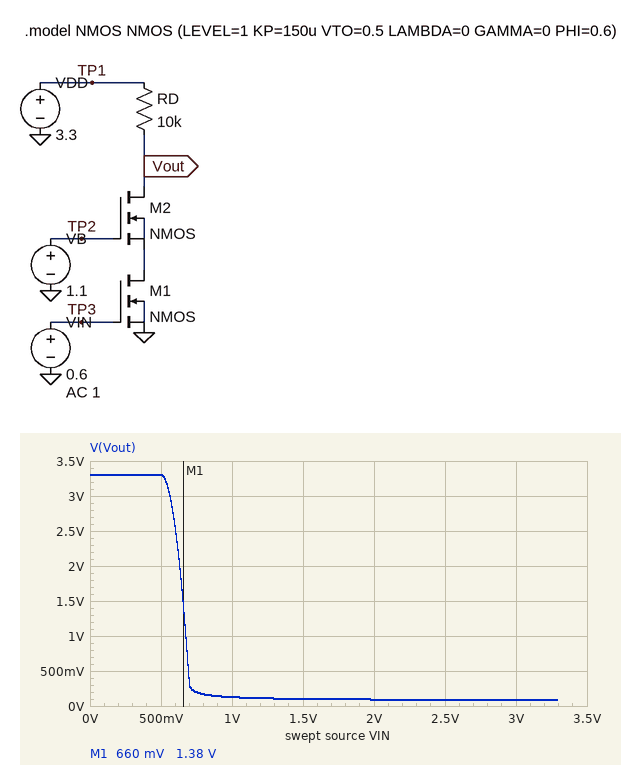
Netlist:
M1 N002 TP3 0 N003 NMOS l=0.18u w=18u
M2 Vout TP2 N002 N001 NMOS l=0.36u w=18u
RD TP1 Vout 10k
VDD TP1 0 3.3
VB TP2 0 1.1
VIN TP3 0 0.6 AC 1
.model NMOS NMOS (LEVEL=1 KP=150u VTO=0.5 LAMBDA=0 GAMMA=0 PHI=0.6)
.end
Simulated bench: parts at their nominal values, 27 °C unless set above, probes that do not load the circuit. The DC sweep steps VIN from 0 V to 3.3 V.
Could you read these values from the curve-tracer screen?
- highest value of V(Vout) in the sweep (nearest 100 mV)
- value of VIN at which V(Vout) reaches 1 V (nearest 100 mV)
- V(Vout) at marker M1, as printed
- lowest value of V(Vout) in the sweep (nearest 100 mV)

3.3 V
700 mV
1.38 V
100 mV
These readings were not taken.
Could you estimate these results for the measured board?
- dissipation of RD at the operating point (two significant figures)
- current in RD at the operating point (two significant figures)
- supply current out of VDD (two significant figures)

56 µW
75 µA
75 µA
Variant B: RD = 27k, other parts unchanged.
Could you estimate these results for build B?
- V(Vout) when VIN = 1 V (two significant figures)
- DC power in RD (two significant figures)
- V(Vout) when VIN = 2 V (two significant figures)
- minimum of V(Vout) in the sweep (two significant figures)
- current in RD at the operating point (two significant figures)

45 mV
150 µW
33 mV
31 mV
75 µA
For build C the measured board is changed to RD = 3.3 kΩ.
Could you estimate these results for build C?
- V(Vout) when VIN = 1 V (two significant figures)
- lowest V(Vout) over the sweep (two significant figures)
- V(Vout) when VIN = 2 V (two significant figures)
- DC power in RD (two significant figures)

560 mV
300 mV
330 mV
19 µW
